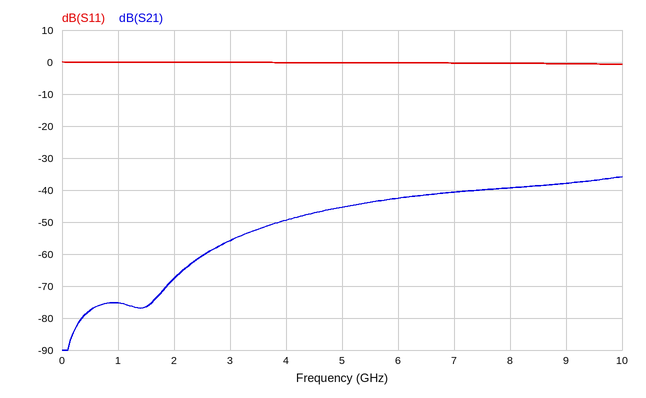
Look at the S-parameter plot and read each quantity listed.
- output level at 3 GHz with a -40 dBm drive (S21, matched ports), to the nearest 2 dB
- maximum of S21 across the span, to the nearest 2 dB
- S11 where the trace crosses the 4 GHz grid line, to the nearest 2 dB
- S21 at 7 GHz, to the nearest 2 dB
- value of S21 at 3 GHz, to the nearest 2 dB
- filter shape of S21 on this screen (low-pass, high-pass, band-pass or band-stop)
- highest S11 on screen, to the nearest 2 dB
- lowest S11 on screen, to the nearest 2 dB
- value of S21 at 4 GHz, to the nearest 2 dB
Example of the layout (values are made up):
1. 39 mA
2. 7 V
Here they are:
1. -96 dBm
2. -36 dB
3. 0 dB
4. -40 dB
5. -56 dB
6. high-pass
7. 0 dB
8. 0 dB
9. -50 dB
